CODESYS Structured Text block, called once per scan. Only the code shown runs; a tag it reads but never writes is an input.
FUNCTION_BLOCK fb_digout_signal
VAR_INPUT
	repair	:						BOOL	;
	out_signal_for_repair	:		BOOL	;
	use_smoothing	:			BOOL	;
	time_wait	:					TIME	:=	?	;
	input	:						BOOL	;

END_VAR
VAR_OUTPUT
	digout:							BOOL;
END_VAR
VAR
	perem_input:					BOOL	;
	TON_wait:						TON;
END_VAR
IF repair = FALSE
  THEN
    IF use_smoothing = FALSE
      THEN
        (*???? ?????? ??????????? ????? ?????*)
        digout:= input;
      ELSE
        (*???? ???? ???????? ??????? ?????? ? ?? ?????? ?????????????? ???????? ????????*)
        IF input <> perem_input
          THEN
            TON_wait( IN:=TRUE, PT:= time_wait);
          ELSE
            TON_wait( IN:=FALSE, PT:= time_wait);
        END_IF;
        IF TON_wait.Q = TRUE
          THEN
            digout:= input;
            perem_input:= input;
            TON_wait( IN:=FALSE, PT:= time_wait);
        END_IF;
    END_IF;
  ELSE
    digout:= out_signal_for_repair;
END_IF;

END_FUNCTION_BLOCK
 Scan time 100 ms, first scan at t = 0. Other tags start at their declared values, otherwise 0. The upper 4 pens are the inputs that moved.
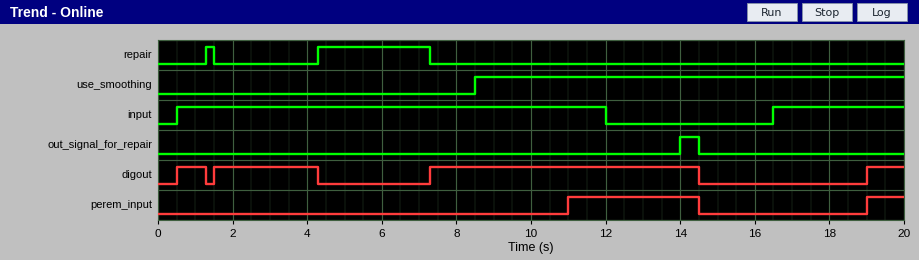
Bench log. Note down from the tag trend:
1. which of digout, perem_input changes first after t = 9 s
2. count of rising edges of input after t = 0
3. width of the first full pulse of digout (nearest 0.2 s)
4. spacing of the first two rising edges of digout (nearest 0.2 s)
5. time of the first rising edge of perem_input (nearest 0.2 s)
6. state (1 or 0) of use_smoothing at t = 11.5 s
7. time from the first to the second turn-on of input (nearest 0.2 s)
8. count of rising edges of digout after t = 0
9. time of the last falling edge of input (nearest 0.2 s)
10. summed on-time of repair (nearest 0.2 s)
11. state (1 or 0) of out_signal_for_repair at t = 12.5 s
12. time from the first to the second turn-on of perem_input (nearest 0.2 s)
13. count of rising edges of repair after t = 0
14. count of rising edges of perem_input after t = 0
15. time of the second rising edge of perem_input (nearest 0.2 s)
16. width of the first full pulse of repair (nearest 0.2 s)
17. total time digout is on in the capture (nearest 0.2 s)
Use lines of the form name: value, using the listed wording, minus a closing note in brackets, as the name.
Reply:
which of digout, perem_input changes first after t = 9 s: perem_input
count of rising edges of input after t = 0: 2
width of the first full pulse of digout: 0.8 s
spacing of the first two rising edges of digout: 1.0 s
time of the first rising edge of perem_input: 11.0 s
state (1 or 0) of use_smoothing at t = 11.5 s: 1
time from the first to the second turn-on of input: 16.0 s
count of rising edges of digout after t = 0: 4
time of the last falling edge of input: 12.0 s
summed on-time of repair: 3.2 s
state (1 or 0) of out_signal_for_repair at t = 12.5 s: 0
time from the first to the second turn-on of perem_input: 8.0 s
count of rising edges of repair after t = 0: 2
count of rising edges of perem_input after t = 0: 2
time of the second rising edge of perem_input: 19.0 s
width of the first full pulse of repair: 0.2 s
total time digout is on in the capture: 11.8 s
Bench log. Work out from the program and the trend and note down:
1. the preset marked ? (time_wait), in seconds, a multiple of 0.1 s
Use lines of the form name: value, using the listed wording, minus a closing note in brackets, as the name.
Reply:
the preset marked ? (time_wait), in seconds, a multiple of 0.1 s: 2.5 s
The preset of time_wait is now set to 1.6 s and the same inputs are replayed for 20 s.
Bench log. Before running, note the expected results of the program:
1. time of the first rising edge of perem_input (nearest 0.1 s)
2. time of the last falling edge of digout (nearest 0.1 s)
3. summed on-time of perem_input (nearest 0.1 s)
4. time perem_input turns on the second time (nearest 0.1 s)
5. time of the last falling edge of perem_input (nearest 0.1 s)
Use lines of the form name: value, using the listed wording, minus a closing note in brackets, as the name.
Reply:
time of the first rising edge of perem_input: 10.1 s
time of the last falling edge of digout: 13.6 s
summed on-time of perem_input: 5.4 s
time perem_input turns on the second time: 18.1 s
time of the last falling edge of perem_input: 13.6 s
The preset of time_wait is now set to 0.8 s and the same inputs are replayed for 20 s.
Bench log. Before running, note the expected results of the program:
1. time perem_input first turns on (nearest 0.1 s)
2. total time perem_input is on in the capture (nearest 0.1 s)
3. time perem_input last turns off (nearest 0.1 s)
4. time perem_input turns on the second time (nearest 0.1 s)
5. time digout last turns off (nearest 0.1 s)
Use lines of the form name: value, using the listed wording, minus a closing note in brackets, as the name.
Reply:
time perem_input first turns on: 9.3 s
total time perem_input is on in the capture: 6.2 s
time perem_input last turns off: 12.8 s
time perem_input turns on the second time: 17.3 s
time digout last turns off: 12.8 s
